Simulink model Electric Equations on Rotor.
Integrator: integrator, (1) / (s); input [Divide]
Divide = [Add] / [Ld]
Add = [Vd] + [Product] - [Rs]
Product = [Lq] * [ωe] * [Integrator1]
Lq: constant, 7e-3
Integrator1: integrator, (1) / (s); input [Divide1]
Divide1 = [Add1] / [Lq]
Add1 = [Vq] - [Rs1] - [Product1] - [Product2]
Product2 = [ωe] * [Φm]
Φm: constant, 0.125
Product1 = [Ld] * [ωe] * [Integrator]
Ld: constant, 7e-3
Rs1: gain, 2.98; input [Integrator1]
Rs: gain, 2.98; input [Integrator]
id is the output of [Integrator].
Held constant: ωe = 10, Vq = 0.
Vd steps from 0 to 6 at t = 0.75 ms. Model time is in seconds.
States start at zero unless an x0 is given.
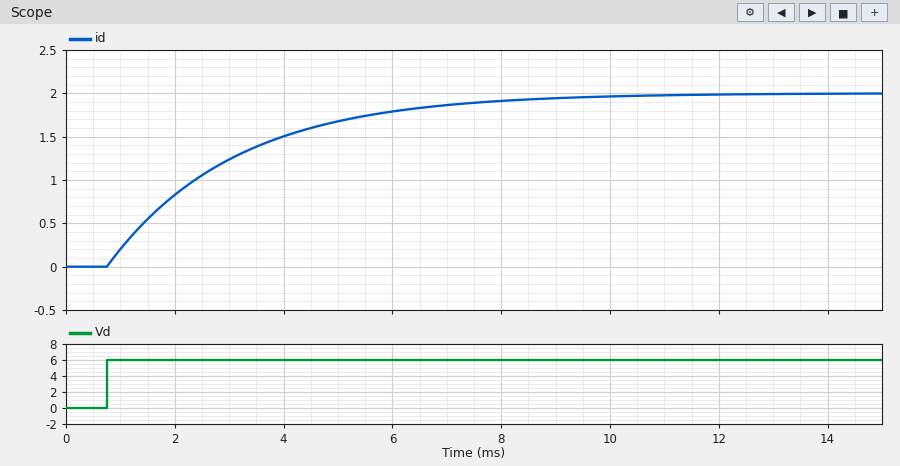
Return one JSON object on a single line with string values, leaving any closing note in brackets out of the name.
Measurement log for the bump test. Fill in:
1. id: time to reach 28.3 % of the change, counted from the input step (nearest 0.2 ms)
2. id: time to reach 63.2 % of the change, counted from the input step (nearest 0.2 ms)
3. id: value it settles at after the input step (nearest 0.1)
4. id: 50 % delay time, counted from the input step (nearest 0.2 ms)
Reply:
{"id: time to reach 28.3 % of the change, counted from the input step": "0.8 ms", "id: time to reach 63.2 % of the change, counted from the input step": "2.4 ms", "id: value it settles at after the input step": "2.0", "id: 50 % delay time, counted from the input step": "1.6 ms"}
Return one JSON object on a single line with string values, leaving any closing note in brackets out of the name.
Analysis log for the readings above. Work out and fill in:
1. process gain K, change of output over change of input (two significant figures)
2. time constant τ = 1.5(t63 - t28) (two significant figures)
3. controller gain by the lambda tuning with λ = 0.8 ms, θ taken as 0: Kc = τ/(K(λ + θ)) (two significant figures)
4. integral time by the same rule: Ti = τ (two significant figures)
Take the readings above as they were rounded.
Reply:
{"process gain K, change of output over change of input": "0.33", "time constant τ = 1.5(t63 - t28)": "2.4 ms", "controller gain by the lambda tuning with λ = 0.8 ms, θ taken as 0: Kc = τ/(K(λ + θ))": "9.1", "integral time by the same rule: Ti = τ": "2.4 ms"}
